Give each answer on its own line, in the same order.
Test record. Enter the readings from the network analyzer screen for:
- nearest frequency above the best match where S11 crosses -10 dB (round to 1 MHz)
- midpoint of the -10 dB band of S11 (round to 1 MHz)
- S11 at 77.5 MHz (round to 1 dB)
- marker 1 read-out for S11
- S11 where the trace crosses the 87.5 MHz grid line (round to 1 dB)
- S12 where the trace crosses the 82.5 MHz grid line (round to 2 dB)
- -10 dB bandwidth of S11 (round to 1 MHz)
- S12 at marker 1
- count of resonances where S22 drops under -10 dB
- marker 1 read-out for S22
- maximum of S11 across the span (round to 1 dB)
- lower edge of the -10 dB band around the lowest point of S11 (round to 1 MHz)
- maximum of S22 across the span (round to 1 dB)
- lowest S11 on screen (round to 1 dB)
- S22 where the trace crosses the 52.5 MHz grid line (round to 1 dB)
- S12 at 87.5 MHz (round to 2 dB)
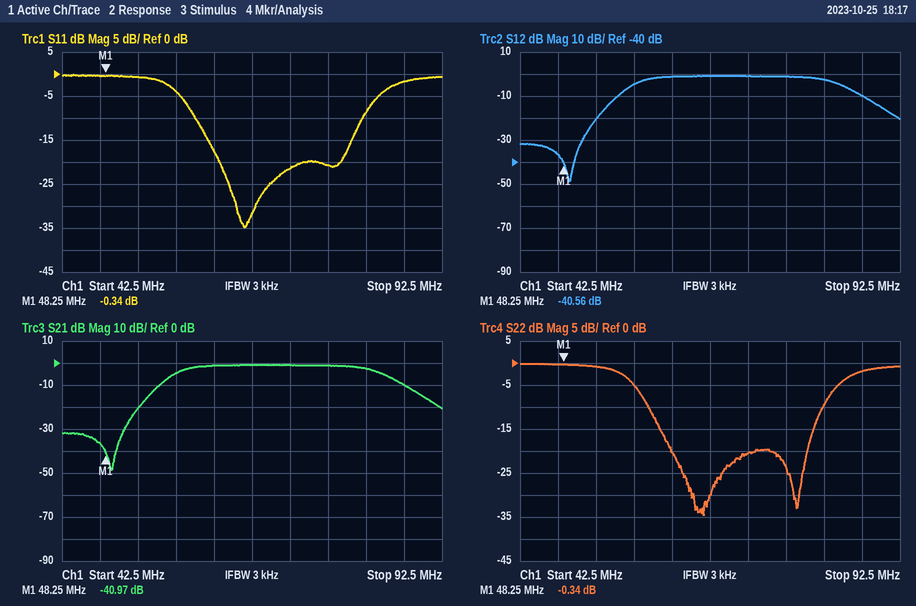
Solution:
82 MHz
71 MHz
-21 dB
-0.34 dB
-2 dB
-2 dB
22 MHz
-40.56 dB
2
-0.34 dB
0 dB
60 MHz
0 dB
-35 dB
-1 dB
-10 dB
